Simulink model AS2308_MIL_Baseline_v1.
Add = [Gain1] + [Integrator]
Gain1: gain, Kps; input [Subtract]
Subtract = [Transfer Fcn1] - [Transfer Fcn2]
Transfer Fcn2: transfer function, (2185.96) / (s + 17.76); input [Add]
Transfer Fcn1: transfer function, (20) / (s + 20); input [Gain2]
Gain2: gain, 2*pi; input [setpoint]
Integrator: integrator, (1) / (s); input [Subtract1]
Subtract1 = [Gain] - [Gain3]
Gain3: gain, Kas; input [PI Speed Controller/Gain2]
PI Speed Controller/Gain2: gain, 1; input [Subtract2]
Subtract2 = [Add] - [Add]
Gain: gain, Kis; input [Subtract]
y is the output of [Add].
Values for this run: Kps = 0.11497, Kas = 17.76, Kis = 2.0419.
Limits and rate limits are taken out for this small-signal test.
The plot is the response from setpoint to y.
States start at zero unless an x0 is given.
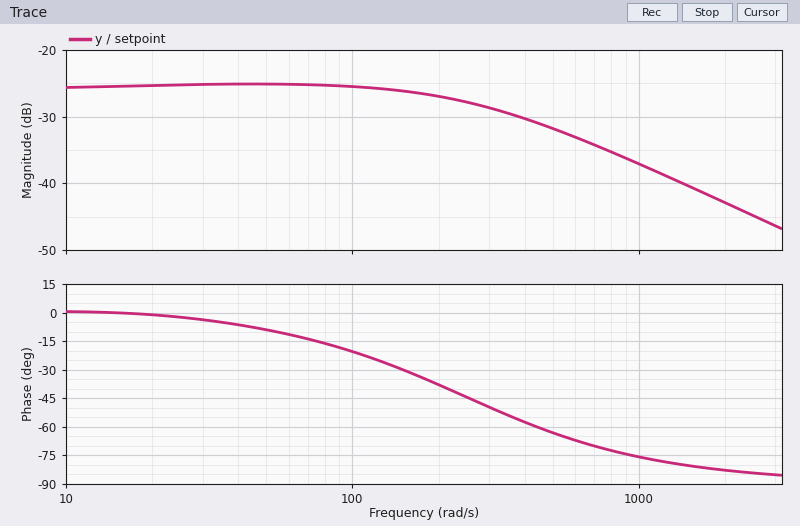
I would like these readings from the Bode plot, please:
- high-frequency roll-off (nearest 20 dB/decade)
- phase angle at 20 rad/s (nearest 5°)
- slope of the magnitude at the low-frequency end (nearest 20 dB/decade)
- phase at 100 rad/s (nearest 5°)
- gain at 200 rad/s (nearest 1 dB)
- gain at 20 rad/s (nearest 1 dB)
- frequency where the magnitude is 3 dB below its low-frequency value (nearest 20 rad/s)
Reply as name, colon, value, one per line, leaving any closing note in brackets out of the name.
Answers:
high-frequency roll-off: -20 dB/decade
phase angle at 20 rad/s: 0°
slope of the magnitude at the low-frequency end: 0 dB/decade
phase at 100 rad/s: -20°
gain at 200 rad/s: -27 dB
gain at 20 rad/s: -25 dB
frequency where the magnitude is 3 dB below its low-frequency value: 300 rad/s
